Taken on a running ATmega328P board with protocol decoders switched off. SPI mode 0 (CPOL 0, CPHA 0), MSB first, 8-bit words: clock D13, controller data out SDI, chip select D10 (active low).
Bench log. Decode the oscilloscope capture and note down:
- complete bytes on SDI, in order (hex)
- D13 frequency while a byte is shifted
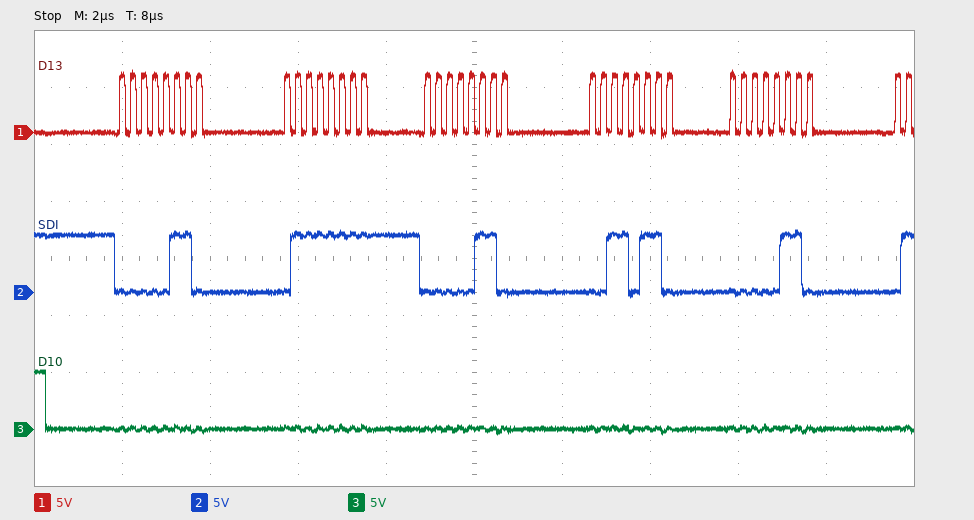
06 7F 06 36 06
4 MHz
